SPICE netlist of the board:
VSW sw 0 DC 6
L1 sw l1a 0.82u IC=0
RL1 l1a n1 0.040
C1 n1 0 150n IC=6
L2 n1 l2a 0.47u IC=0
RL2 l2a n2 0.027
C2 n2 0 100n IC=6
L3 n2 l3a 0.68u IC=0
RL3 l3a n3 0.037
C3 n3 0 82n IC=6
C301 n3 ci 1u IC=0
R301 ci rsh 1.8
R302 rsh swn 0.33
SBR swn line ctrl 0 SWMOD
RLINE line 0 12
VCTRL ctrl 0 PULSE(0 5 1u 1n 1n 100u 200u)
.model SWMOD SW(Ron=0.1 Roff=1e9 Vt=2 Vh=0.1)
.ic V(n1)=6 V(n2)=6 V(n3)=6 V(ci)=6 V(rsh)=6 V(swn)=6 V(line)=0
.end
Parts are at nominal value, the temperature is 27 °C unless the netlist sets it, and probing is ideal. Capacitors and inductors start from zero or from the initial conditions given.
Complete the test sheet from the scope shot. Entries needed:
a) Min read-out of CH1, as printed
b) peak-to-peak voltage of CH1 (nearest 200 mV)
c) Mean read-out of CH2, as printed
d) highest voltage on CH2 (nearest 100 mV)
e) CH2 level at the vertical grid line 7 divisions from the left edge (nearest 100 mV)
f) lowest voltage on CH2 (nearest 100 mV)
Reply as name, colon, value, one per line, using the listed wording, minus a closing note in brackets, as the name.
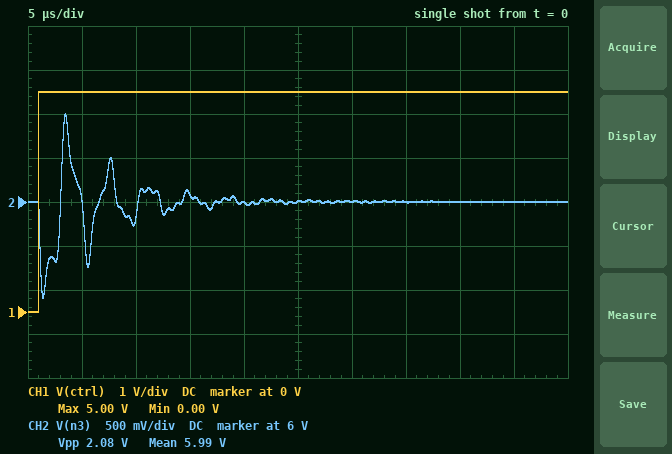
Min read-out of CH1, as printed: 0.00 V
peak-to-peak voltage of CH1: 5.0 V
Mean read-out of CH2, as printed: 5.99 V
highest voltage on CH2: 7.0 V
CH2 level at the vertical grid line 7 divisions from the left edge: 6.0 V
lowest voltage on CH2: 4.9 V
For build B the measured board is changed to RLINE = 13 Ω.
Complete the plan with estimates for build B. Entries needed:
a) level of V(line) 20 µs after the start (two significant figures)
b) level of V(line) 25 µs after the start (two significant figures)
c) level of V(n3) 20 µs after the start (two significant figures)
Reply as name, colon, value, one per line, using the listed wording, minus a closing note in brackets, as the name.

level of V(line) 20 µs after the start: 1.5 V
level of V(line) 25 µs after the start: 1.1 V
level of V(n3) 20 µs after the start: 6.0 V
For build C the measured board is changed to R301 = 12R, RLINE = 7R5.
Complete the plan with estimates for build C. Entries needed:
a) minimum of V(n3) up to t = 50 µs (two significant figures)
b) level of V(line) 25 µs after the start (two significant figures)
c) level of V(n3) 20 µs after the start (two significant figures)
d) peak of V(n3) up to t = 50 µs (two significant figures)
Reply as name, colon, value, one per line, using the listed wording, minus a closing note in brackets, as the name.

minimum of V(n3) up to t = 50 µs: 5.2 V
level of V(line) 25 µs after the start: 680 mV
level of V(n3) 20 µs after the start: 6.0 V
peak of V(n3) up to t = 50 µs: 6.8 V
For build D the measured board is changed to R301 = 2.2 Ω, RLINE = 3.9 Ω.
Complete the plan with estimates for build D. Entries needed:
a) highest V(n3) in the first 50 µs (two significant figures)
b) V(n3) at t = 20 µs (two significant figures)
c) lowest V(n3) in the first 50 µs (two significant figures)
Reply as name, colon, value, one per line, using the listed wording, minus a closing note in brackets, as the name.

highest V(n3) in the first 50 µs: 7.4 V
V(n3) at t = 20 µs: 6.0 V
lowest V(n3) in the first 50 µs: 4.0 V
